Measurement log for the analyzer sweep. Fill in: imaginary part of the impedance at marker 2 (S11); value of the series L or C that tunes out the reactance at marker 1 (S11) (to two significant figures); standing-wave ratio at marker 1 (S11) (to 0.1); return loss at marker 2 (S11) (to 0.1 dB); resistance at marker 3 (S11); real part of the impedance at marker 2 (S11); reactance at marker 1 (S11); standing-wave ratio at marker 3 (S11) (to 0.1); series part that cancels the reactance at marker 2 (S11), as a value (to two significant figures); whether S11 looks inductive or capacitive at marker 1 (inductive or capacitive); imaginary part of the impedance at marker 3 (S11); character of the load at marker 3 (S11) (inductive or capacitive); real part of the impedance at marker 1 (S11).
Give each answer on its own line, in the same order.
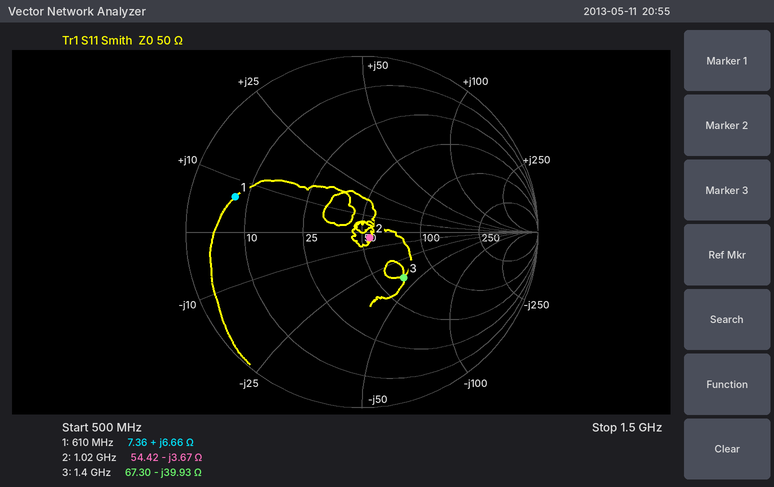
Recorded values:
-3.67 Ω
39 pF
6.9
25.2 dB
67.30 Ω
54.42 Ω
+6.66 Ω
2.1
570 pH
inductive
-39.93 Ω
capacitive
7.36 Ω
